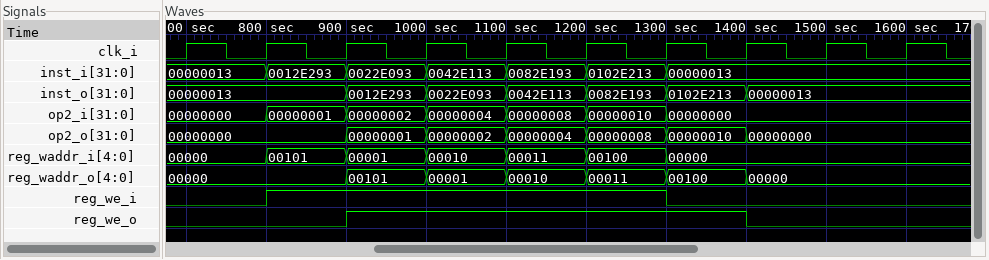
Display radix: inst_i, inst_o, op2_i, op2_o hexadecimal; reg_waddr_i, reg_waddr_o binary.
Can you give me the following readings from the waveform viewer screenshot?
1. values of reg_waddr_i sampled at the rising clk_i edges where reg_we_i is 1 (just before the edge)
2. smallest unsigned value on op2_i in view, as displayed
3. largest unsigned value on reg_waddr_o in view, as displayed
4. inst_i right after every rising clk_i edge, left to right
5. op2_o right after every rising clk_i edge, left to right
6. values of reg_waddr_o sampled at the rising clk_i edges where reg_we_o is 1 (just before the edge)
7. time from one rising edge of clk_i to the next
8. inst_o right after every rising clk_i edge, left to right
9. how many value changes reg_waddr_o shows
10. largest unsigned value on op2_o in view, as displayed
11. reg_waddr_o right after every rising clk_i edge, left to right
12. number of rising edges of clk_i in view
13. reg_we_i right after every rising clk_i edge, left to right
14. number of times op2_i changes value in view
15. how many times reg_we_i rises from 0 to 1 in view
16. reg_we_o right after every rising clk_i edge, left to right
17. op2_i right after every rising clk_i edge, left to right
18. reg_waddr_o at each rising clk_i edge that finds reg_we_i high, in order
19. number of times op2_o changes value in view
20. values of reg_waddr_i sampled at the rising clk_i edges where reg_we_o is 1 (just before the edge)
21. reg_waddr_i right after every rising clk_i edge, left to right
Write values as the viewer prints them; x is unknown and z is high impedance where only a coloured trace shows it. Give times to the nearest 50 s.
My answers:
00101, 00001, 00010, 00011, 00100
00000000
00101
00000013, 0012E293, 0022E093, 0042E113, 0082E193, 0102E213, 00000013, 00000013, 00000013, 00000013
00000000, 00000000, 00000001, 00000002, 00000004, 00000008, 00000010, 00000000, 00000000, 00000000
00101, 00001, 00010, 00011, 00100
100 s
00000013, 00000013, 0012E293, 0022E093, 0042E113, 0082E193, 0102E213, 00000013, 00000013, 00000013
6
00000010
00000, 00000, 00101, 00001, 00010, 00011, 00100, 00000, 00000, 00000
10
0 1 1 1 1 1 0 0 0 0
6
1
0 0 1 1 1 1 1 0 0 0
00000000, 00000001, 00000002, 00000004, 00000008, 00000010, 00000000, 00000000, 00000000, 00000000
00000, 00101, 00001, 00010, 00011
6
00001, 00010, 00011, 00100, 00000
00000, 00101, 00001, 00010, 00011, 00100, 00000, 00000, 00000, 00000
